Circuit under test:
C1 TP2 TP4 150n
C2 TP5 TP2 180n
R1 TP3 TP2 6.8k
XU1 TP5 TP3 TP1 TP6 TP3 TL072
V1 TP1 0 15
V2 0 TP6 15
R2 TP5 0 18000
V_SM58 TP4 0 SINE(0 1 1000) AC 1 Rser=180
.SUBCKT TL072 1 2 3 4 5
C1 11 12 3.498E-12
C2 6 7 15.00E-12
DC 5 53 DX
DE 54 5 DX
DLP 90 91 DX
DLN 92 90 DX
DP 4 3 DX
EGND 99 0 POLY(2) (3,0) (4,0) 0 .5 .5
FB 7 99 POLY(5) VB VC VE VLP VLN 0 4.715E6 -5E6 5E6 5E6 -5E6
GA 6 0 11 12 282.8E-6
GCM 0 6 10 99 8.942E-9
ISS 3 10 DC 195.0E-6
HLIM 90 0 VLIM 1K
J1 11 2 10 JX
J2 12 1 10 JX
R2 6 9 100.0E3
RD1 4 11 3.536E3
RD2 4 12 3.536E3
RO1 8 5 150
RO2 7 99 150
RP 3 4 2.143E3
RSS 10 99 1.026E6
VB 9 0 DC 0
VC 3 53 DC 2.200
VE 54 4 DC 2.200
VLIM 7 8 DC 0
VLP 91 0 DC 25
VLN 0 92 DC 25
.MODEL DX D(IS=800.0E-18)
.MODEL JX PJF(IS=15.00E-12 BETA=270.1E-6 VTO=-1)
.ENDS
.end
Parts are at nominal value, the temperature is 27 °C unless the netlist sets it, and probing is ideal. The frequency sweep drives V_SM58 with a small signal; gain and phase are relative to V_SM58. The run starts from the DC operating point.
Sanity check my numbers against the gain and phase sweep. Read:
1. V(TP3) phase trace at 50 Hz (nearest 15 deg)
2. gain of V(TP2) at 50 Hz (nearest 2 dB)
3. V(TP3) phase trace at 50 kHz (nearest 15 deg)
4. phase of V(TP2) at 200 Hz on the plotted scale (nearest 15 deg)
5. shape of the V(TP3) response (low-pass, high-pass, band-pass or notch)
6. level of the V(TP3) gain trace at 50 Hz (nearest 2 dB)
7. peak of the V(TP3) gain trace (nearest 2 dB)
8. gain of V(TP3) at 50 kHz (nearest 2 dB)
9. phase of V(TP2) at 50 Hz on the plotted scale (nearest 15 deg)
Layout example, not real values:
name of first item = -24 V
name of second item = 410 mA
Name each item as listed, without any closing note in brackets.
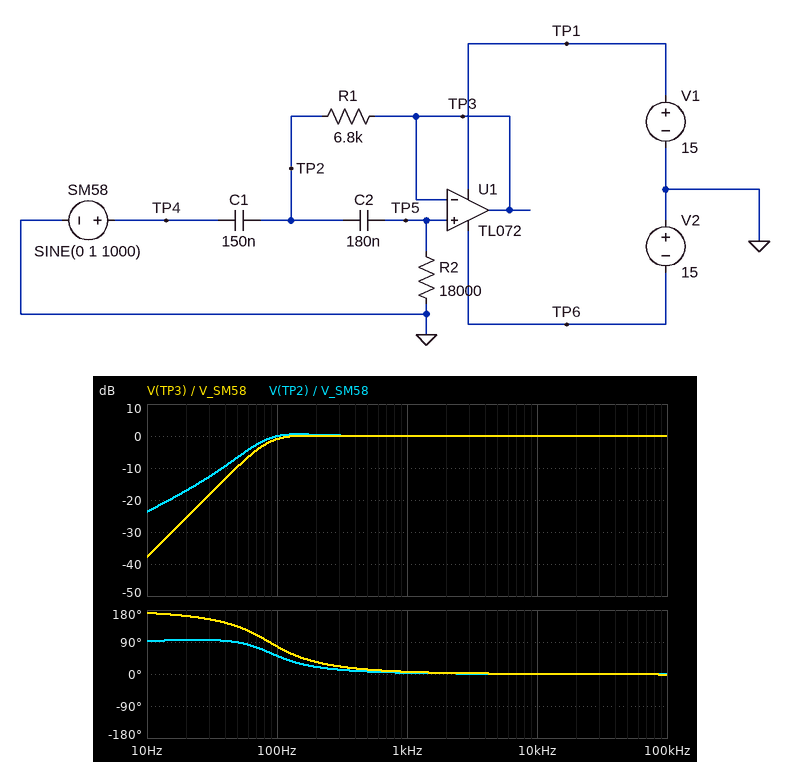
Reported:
V(TP3) phase trace at 50 Hz = 135 deg
gain of V(TP2) at 50 Hz = -6 dB
V(TP3) phase trace at 50 kHz = 0 deg
phase of V(TP2) at 200 Hz on the plotted scale = 15 deg
shape of the V(TP3) response = high-pass
level of the V(TP3) gain trace at 50 Hz = -10 dB
peak of the V(TP3) gain trace = 0 dB
gain of V(TP3) at 50 kHz = 0 dB
phase of V(TP2) at 50 Hz on the plotted scale = 90 deg
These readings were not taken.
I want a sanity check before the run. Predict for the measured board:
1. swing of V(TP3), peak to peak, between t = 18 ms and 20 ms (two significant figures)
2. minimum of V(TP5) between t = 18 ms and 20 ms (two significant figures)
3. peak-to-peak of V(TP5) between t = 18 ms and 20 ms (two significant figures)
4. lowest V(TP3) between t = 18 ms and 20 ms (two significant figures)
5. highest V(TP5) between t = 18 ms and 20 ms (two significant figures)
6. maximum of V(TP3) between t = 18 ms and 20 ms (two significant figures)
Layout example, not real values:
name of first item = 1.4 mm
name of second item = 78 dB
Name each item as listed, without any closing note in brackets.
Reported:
swing of V(TP3), peak to peak, between t = 18 ms and 20 ms = 2.0 V
minimum of V(TP5) between t = 18 ms and 20 ms = -990 mV
peak-to-peak of V(TP5) between t = 18 ms and 20 ms = 2.0 V
lowest V(TP3) between t = 18 ms and 20 ms = -990 mV
highest V(TP5) between t = 18 ms and 20 ms = 990 mV
maximum of V(TP3) between t = 18 ms and 20 ms = 990 mV
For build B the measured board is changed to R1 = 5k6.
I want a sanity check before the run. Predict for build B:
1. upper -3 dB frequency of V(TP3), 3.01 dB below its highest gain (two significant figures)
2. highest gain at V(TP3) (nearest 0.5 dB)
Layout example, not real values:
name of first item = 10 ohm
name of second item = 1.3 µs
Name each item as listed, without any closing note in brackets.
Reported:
upper -3 dB frequency of V(TP3), 3.01 dB below its highest gain = 4.2 MHz
highest gain at V(TP3) = 0.5 dB
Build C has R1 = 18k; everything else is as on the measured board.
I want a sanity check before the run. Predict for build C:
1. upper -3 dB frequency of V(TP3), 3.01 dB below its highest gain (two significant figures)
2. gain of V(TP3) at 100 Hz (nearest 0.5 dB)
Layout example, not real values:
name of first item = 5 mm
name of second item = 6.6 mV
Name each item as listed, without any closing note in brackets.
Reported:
upper -3 dB frequency of V(TP3), 3.01 dB below its highest gain = 4.7 MHz
gain of V(TP3) at 100 Hz = -2.5 dB
